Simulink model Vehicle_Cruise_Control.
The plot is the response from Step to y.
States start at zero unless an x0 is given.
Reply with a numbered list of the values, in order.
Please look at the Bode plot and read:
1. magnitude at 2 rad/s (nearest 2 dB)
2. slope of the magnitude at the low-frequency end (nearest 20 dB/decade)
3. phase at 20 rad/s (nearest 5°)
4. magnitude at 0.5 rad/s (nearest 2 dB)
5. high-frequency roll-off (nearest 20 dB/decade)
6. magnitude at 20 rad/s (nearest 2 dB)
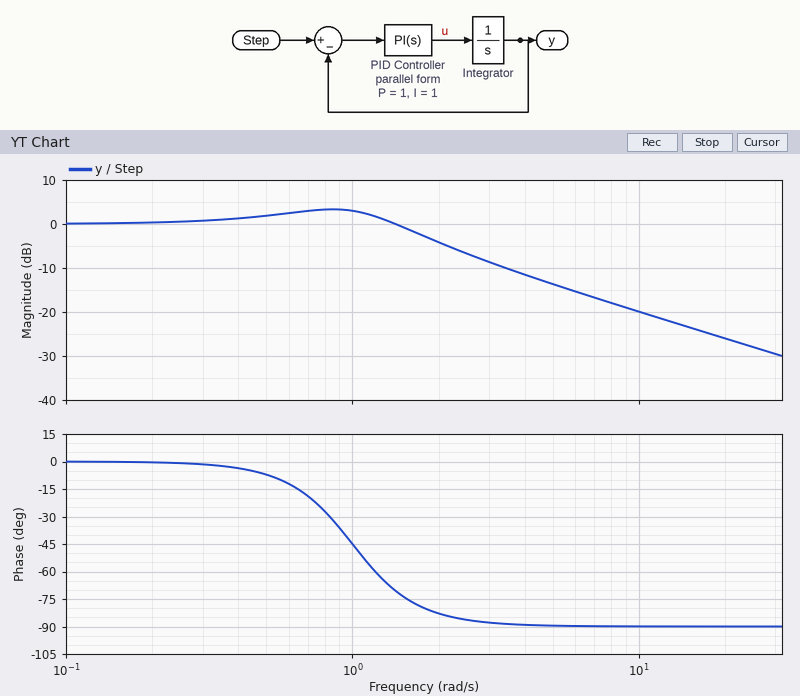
1. -4 dB
2. 0 dB/decade
3. -90°
4. 2 dB
5. -20 dB/decade
6. -26 dB
